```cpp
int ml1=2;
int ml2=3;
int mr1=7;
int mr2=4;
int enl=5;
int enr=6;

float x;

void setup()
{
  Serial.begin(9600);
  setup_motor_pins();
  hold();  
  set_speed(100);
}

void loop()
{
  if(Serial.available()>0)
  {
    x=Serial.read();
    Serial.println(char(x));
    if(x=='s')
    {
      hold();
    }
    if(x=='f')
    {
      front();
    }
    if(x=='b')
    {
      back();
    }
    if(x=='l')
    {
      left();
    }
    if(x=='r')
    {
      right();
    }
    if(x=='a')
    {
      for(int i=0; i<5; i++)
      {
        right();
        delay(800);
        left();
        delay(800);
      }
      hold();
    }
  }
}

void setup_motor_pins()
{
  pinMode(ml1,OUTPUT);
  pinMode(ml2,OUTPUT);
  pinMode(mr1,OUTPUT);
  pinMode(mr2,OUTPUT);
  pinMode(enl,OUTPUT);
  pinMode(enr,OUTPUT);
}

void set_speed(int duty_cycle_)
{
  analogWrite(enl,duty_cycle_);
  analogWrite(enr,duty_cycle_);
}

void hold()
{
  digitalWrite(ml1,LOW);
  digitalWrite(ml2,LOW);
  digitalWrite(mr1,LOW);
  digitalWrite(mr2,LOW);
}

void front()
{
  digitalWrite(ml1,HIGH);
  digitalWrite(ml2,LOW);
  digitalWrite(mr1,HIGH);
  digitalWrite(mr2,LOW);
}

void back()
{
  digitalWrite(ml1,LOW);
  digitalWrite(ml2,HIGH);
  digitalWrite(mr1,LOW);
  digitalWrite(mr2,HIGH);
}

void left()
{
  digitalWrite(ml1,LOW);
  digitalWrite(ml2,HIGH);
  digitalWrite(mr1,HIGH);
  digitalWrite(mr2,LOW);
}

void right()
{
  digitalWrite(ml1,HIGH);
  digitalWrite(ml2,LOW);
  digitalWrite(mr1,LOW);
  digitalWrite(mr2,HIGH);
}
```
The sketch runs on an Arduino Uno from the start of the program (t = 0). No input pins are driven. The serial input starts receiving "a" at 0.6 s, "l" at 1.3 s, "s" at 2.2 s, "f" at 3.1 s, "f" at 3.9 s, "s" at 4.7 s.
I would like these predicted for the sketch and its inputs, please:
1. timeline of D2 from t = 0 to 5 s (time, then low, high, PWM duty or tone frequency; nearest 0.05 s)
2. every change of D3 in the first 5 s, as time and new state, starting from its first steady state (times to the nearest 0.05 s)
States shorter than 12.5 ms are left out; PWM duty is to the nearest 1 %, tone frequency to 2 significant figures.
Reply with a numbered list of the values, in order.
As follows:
1. 0 s low; 0.6 s high; 1.4 s low; 2.2 s high; 3 s low; 3.8 s high; 4.6 s low
2. 0 s low; 1.4 s high; 2.2 s low; 3 s high; 3.8 s low; 4.6 s high
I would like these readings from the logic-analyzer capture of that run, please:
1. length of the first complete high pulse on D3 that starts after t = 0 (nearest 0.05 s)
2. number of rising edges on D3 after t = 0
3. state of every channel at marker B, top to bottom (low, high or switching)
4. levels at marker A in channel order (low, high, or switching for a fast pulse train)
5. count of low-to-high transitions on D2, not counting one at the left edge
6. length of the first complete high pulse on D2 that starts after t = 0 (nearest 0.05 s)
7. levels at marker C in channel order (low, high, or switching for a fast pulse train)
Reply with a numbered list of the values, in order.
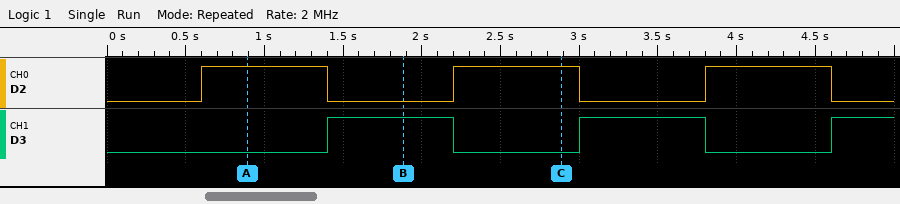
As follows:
1. 0.80 s
2. 3
3. D2 low, D3 high
4. D2 high, D3 low
5. 3
6. 0.80 s
7. D2 high, D3 low
